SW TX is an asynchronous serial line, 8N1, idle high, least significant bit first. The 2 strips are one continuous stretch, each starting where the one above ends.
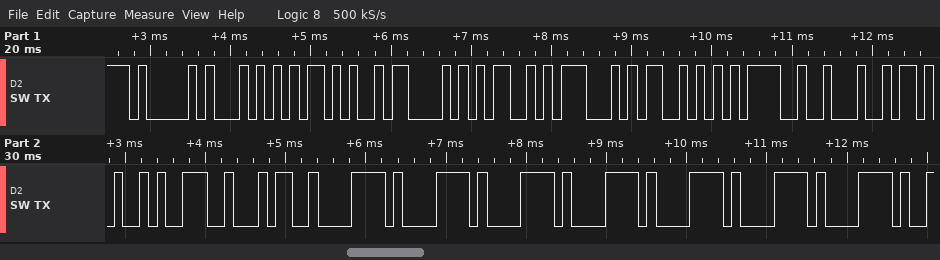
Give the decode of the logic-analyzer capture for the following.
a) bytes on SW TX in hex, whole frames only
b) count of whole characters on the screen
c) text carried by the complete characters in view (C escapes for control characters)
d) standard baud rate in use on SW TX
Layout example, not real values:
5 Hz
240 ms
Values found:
41 54 2B 43 4D 47 53 3D 22 2B 39 34 78 78 78 78 78 78 78
19
"AT+CMGS=\"+94xxxxxxx"
9600 baud
